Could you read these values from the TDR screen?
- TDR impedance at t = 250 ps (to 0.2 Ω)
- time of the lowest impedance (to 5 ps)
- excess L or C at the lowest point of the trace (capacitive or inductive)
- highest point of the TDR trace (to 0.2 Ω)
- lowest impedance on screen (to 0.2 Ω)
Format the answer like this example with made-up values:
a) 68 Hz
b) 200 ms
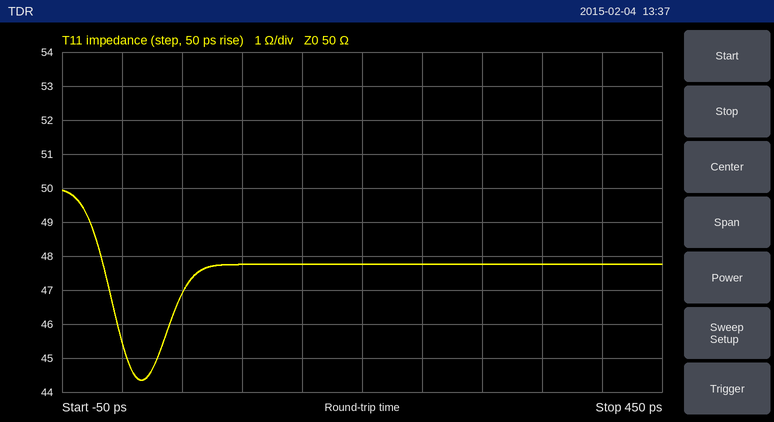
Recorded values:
a) 47.8 Ω
b) 15 ps
c) capacitive
d) 50.0 Ω
e) 44.4 Ω
